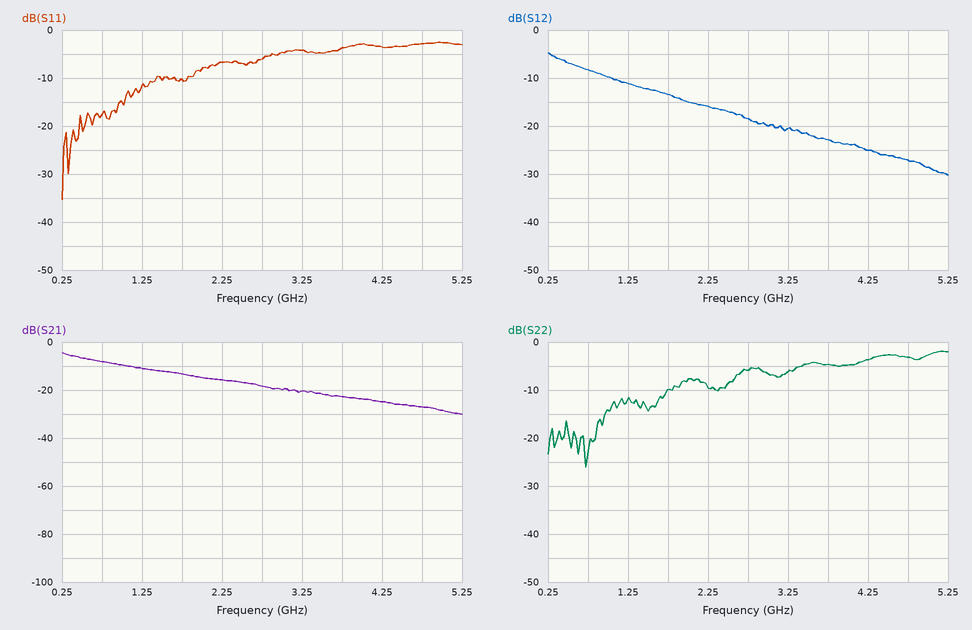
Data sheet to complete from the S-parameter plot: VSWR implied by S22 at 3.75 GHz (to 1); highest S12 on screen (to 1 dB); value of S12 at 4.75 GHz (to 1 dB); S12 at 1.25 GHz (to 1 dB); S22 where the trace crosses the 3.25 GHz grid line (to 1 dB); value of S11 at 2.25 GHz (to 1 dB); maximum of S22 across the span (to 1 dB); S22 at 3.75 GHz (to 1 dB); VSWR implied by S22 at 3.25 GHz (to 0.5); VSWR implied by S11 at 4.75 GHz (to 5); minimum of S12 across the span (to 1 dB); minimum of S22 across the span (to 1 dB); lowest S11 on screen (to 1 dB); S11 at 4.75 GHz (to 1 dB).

4
-5 dB
-27 dB
-11 dB
-6 dB
-7 dB
-2 dB
-5 dB
3.0
5
-30 dB
-26 dB
-35 dB
-3 dB
